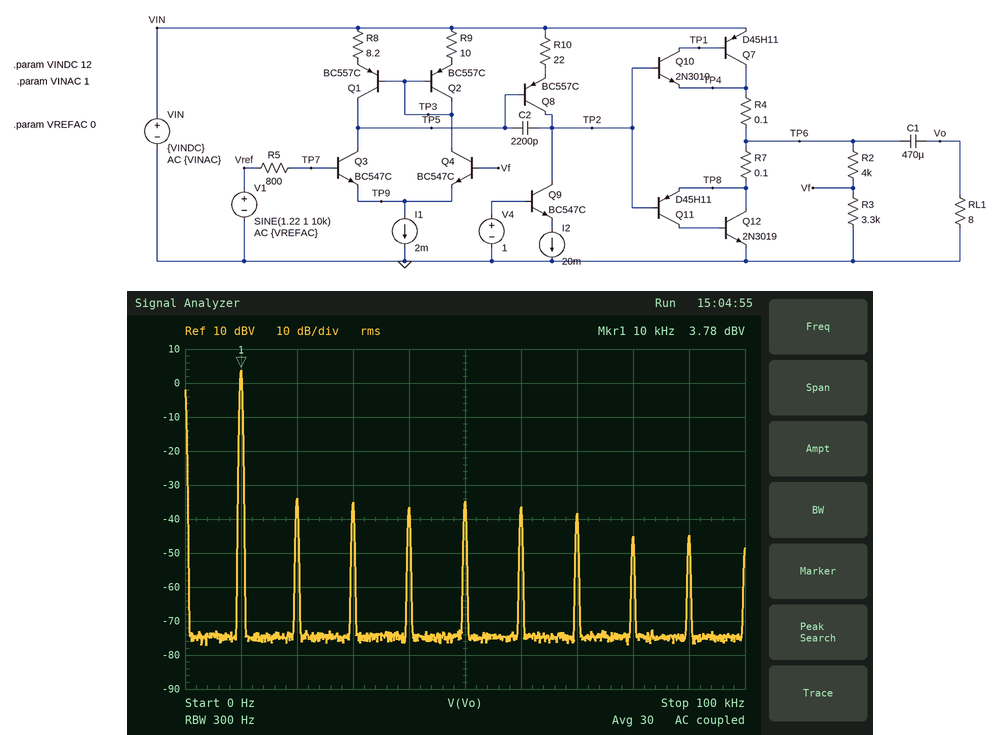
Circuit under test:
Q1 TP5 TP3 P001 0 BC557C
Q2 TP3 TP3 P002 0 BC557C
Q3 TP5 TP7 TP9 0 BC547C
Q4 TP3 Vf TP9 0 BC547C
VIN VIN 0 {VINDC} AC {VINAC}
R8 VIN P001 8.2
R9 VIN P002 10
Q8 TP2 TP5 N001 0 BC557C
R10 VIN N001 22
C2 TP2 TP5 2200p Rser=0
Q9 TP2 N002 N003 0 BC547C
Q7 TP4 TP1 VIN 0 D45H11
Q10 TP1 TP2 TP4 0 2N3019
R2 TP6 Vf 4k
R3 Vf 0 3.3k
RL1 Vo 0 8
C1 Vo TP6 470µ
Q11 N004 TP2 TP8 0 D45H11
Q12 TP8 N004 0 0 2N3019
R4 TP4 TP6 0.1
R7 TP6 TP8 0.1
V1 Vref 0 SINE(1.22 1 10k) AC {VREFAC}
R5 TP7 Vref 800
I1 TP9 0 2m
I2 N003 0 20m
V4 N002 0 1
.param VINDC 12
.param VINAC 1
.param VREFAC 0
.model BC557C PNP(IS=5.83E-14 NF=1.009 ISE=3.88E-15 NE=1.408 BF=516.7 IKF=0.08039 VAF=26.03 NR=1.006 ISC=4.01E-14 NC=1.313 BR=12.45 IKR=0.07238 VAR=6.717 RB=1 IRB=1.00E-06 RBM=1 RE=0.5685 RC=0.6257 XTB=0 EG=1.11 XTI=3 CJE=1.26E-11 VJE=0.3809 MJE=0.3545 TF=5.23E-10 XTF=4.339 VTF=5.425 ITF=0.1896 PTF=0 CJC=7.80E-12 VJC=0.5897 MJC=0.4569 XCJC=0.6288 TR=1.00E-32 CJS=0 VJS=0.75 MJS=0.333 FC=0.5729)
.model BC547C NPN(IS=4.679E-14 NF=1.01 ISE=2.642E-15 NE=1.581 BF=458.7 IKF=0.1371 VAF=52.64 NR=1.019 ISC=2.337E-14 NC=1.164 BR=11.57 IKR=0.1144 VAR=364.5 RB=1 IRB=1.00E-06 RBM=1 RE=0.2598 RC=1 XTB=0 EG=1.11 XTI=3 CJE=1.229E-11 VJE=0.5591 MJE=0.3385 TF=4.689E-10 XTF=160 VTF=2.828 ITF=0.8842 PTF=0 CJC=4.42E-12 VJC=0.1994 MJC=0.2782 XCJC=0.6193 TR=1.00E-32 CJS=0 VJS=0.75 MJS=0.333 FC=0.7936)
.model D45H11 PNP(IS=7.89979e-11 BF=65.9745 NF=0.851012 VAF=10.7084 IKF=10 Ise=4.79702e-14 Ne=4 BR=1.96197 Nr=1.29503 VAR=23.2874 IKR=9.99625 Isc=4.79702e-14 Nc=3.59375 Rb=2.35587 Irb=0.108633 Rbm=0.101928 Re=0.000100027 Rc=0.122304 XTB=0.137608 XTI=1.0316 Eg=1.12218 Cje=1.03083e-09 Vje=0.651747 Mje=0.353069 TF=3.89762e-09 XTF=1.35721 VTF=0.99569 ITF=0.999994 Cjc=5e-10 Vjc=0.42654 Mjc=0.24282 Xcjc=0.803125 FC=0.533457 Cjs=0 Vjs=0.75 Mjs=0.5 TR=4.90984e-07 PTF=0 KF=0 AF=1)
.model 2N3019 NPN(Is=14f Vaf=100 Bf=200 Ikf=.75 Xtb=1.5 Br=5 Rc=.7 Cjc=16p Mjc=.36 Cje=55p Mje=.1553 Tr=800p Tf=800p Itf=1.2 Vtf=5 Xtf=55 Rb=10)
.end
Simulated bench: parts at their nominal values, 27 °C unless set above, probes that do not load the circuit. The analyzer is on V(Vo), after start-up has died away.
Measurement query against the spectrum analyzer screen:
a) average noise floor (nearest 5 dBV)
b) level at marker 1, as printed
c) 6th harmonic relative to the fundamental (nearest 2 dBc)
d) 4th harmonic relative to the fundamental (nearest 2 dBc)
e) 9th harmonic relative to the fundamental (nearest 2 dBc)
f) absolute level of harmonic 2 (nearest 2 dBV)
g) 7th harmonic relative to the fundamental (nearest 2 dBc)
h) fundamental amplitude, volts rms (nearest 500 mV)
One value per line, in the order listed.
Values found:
-75 dBV
3.78 dBV
-40 dBc
-40 dBc
-48 dBc
-34 dBV
-42 dBc
1.5 V
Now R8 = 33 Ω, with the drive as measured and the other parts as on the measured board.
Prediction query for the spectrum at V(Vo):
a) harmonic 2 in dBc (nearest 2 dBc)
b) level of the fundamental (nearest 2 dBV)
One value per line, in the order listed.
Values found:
-42 dBc
4 dBV
